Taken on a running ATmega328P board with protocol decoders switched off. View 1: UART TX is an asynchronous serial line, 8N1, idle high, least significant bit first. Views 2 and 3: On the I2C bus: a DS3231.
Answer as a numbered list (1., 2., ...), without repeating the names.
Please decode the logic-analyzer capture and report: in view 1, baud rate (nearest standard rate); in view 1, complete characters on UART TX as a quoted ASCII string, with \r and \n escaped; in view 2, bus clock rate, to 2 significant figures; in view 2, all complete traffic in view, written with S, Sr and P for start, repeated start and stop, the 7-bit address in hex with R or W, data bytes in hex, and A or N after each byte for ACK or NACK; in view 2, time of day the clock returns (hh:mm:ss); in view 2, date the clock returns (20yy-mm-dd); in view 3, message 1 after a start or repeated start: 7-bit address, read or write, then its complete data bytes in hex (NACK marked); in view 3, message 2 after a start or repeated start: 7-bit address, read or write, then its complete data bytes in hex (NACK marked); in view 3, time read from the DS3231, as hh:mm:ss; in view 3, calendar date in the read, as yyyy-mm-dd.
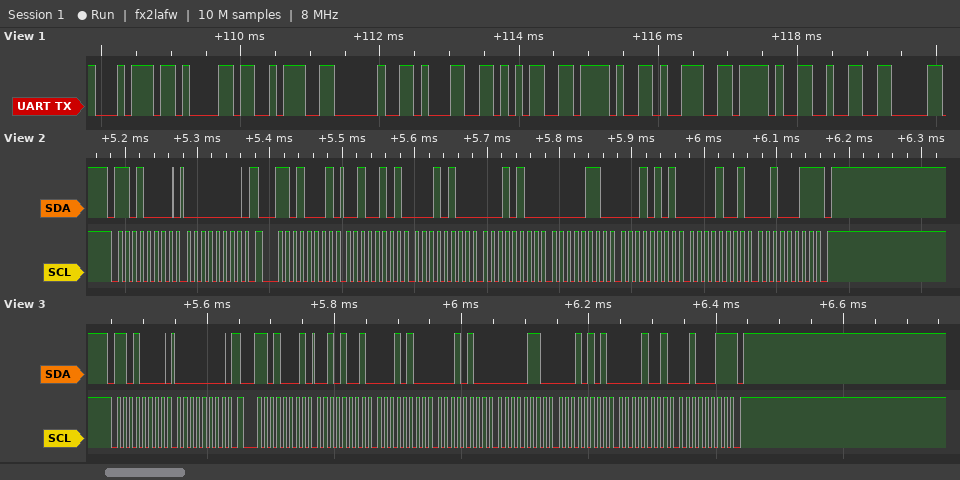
1. 9600 baud
2. "ta: 15/9/2"
3. 100 kHz
4. S 68W A 00 A Sr 68R A 25 A 14 A 14 A 06 A 15 A 09 A 23 N P
5. 14:14:25
6. 2023-09-15
7. 0x68 write: 00
8. 0x68 read: 29 14 14 06 15 09 23 NACK
9. 14:14:29
10. 2023-09-15
